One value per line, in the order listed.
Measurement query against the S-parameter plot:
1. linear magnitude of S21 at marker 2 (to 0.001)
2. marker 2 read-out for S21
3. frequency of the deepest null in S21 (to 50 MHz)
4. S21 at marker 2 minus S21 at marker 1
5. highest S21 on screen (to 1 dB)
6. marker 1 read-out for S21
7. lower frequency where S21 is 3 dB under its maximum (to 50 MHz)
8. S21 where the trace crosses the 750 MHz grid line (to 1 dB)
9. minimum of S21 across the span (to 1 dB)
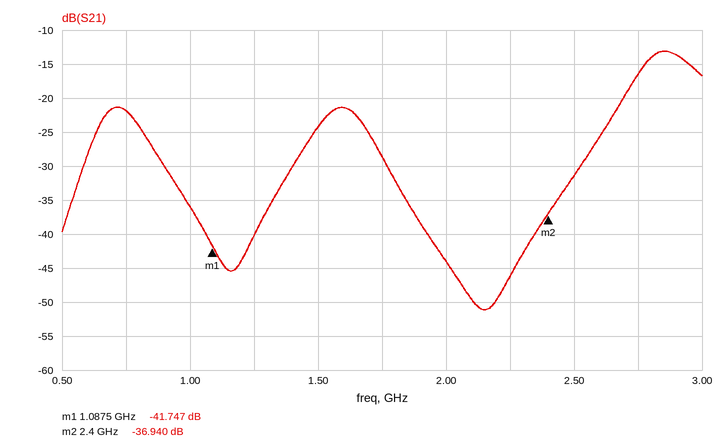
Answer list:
0.014
-36.940 dB
2.15 GHz
4.807 dB
-13 dB
-41.747 dB
2.75 GHz
-22 dB
-51 dB
